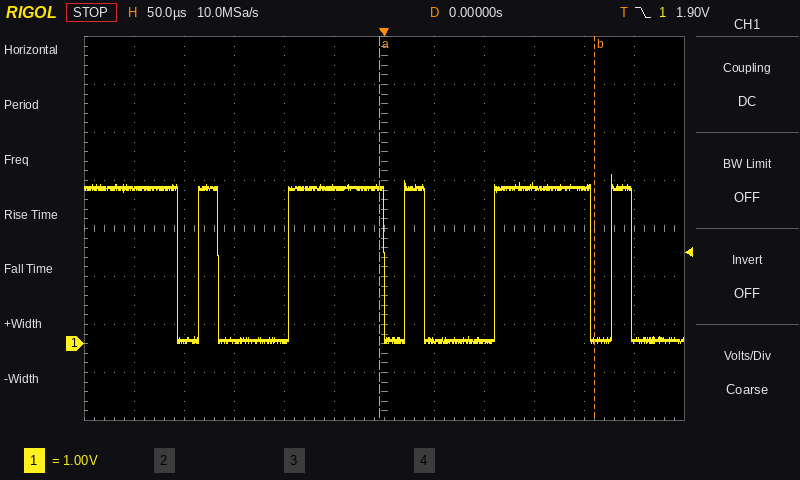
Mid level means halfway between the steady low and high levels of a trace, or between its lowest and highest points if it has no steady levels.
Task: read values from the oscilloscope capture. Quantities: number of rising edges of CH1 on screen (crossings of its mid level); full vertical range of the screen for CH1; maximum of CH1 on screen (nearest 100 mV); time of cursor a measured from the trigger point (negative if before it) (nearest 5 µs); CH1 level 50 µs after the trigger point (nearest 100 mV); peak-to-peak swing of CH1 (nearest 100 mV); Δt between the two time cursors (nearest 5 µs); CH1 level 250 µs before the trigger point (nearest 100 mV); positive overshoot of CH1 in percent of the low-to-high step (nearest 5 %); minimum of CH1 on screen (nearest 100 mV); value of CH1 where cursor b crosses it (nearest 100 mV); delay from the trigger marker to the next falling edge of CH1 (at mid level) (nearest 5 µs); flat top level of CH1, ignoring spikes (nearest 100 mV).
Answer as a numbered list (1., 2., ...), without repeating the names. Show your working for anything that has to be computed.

1. 5
2. 8 V
3. 3.5 V
4. -5 µs
5. 100 mV
6. 3.5 V − (0.0 V) = 3.5 V
7. 215 µs
8. 3.2 V
9. 10 %
10. 0.0 V
11. 100 mV
12. 40 µs
13. 3.2 V
